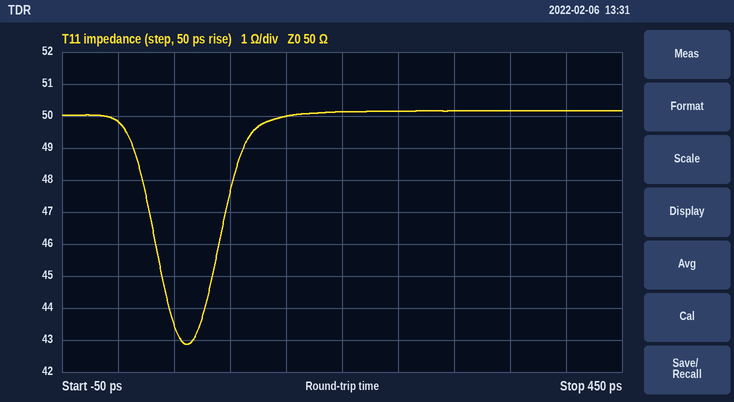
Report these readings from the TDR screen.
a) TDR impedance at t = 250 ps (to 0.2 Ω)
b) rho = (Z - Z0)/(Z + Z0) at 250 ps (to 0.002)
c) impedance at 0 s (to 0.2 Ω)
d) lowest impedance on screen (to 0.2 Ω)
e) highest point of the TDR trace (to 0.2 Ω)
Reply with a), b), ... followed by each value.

a) 50.2 Ω
b) +0.002
c) 49.8 Ω
d) 42.8 Ω
e) 50.2 Ω
